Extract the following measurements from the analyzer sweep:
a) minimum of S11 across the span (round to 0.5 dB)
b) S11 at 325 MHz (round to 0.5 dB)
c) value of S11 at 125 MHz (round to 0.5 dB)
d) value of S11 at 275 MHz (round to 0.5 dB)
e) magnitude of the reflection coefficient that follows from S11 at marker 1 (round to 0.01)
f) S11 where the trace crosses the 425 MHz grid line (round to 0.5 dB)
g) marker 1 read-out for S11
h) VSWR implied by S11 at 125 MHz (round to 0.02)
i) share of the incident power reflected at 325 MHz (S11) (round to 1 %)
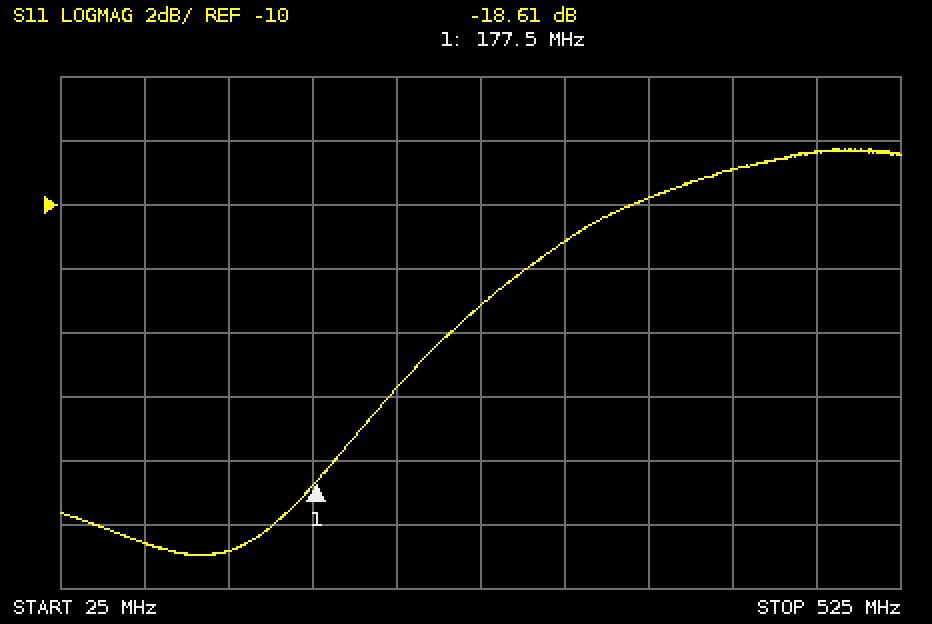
-21.0 dB
-11.0 dB
-21.0 dB
-13.0 dB
0.12
-9.0 dB
-18.61 dB
1.20
8 %
